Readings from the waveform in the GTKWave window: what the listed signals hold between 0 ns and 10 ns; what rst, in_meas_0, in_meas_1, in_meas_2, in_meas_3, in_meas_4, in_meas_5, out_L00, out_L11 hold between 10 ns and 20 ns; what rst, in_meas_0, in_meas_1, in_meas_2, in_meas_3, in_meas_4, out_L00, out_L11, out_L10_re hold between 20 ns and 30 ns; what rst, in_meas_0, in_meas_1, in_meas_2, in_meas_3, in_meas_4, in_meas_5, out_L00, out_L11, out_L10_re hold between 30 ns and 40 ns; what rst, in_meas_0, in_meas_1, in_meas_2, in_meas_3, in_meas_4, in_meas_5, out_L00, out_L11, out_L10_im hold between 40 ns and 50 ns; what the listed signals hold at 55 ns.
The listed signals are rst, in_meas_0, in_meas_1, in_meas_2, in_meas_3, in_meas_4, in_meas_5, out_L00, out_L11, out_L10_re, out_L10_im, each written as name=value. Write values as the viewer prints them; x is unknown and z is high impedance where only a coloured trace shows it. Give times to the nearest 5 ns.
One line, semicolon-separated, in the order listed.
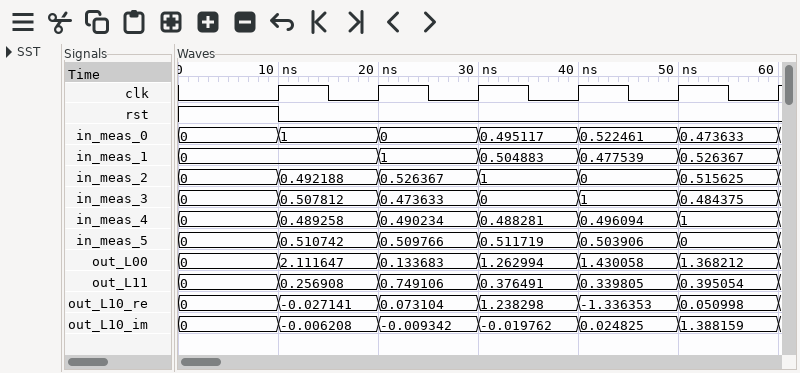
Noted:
rst=1, in_meas_0=0, in_meas_1=0, in_meas_2=0, in_meas_3=0, in_meas_4=0, in_meas_5=0, out_L00=0, out_L11=0, out_L10_re=0, out_L10_im=0; rst=0, in_meas_0=1, in_meas_1=0, in_meas_2=0.492188, in_meas_3=0.507812, in_meas_4=0.489258, in_meas_5=0.510742, out_L00=2.111647, out_L11=0.256908; rst=0, in_meas_0=0, in_meas_1=1, in_meas_2=0.526367, in_meas_3=0.473633, in_meas_4=0.490234, out_L00=0.133683, out_L11=0.749106, out_L10_re=0.073104; rst=0, in_meas_0=0.495117, in_meas_1=0.504883, in_meas_2=1, in_meas_3=0, in_meas_4=0.488281, in_meas_5=0.511719, out_L00=1.262994, out_L11=0.376491, out_L10_re=1.238298; rst=0, in_meas_0=0.522461, in_meas_1=0.477539, in_meas_2=0, in_meas_3=1, in_meas_4=0.496094, in_meas_5=0.503906, out_L00=1.430058, out_L11=0.339805, out_L10_im=0.024825; rst=0, in_meas_0=0.473633, in_meas_1=0.526367, in_meas_2=0.515625, in_meas_3=0.484375, in_meas_4=1, in_meas_5=0, out_L00=1.368212, out_L11=0.395054, out_L10_re=0.050998, out_L10_im=1.388159
